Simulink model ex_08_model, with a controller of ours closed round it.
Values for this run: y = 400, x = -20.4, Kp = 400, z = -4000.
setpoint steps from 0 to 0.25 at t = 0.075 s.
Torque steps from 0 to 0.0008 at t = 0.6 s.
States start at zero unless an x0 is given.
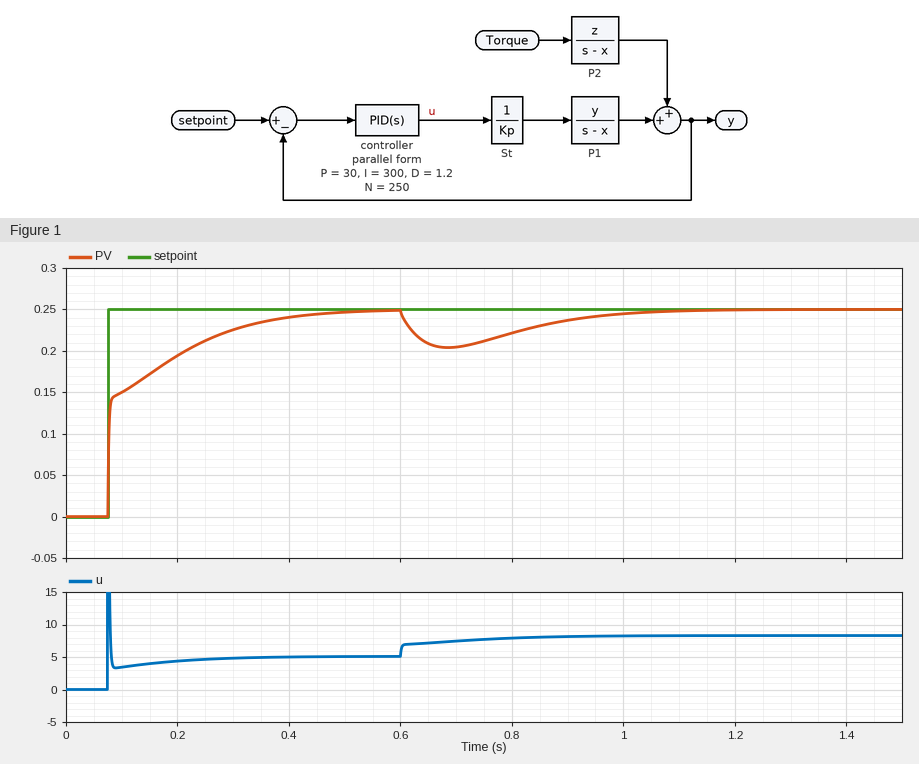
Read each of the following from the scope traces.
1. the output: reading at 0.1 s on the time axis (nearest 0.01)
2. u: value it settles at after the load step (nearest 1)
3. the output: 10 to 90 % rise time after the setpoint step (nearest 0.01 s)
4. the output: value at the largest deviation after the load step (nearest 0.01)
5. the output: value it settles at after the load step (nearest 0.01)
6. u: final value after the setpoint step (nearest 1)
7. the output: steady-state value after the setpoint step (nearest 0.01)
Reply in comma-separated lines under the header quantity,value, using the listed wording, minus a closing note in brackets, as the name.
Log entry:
quantity,value
the output: reading at 0.1 s on the time axis,0.15
u: value it settles at after the load step,8
the output: 10 to 90 % rise time after the setpoint step,0.22 s
the output: value at the largest deviation after the load step,0.20
the output: value it settles at after the load step,0.25
u: final value after the setpoint step,5
the output: steady-state value after the setpoint step,0.25
